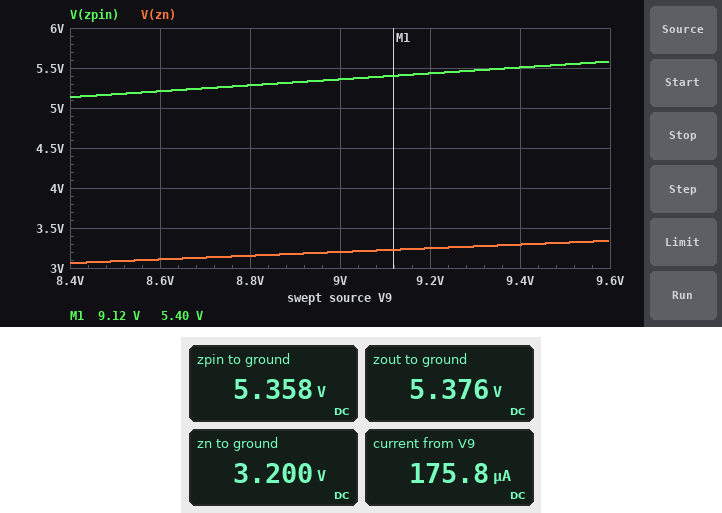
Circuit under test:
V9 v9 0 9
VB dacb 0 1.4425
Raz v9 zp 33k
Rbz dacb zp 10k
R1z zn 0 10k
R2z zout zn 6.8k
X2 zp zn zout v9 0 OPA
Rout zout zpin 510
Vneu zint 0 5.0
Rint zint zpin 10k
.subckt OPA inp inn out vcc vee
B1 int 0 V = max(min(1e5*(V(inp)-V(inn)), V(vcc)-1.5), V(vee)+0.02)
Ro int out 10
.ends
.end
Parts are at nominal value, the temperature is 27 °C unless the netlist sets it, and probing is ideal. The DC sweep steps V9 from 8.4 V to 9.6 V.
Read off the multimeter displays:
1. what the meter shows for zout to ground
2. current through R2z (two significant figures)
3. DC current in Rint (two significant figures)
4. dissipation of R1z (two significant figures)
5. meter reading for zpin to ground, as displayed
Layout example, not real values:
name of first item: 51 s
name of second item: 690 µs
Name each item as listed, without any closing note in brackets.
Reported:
what the meter shows for zout to ground: 5.376 V
current through R2z: 320 µA
DC current in Rint: 36 µA
dissipation of R1z: 1.0 mW
meter reading for zpin to ground, as displayed: 5.358 V
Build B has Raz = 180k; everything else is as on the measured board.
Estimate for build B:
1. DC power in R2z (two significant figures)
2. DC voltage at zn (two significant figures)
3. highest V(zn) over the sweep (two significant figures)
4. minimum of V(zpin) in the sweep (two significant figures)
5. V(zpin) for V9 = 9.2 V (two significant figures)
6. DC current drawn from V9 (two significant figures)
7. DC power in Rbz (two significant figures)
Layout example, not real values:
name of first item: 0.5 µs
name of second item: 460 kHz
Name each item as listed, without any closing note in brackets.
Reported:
DC power in R2z: 230 µW
DC voltage at zn: 1.8 V
highest V(zn) over the sweep: 1.9 V
minimum of V(zpin) in the sweep: 3.1 V
V(zpin) for V9 = 9.2 V: 3.2 V
DC current drawn from V9: 40 µA
DC power in Rbz: 16 µW
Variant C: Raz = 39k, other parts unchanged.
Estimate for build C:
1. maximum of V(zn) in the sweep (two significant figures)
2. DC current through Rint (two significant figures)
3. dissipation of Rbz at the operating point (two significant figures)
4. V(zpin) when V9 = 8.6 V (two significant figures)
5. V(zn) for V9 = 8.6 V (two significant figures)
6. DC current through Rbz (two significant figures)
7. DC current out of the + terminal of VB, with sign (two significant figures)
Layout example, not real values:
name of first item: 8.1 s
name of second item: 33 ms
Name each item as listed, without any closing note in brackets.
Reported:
maximum of V(zn) in the sweep: 3.1 V
DC current through Rint: 1.4 µA
dissipation of Rbz at the operating point: 240 µW
V(zpin) when V9 = 8.6 V: 4.9 V
V(zn) for V9 = 8.6 V: 2.9 V
DC current through Rbz: 150 µA
DC current out of the + terminal of VB, with sign: -150 µA
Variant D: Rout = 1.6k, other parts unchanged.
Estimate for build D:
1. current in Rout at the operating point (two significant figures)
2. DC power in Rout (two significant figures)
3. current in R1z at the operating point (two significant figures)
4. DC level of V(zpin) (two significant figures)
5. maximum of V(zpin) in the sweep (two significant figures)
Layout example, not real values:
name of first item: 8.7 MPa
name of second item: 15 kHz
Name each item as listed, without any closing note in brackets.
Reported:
current in Rout at the operating point: 32 µA
DC power in Rout: 1.7 µW
current in R1z at the operating point: 320 µA
DC level of V(zpin): 5.3 V
maximum of V(zpin) in the sweep: 5.5 V
